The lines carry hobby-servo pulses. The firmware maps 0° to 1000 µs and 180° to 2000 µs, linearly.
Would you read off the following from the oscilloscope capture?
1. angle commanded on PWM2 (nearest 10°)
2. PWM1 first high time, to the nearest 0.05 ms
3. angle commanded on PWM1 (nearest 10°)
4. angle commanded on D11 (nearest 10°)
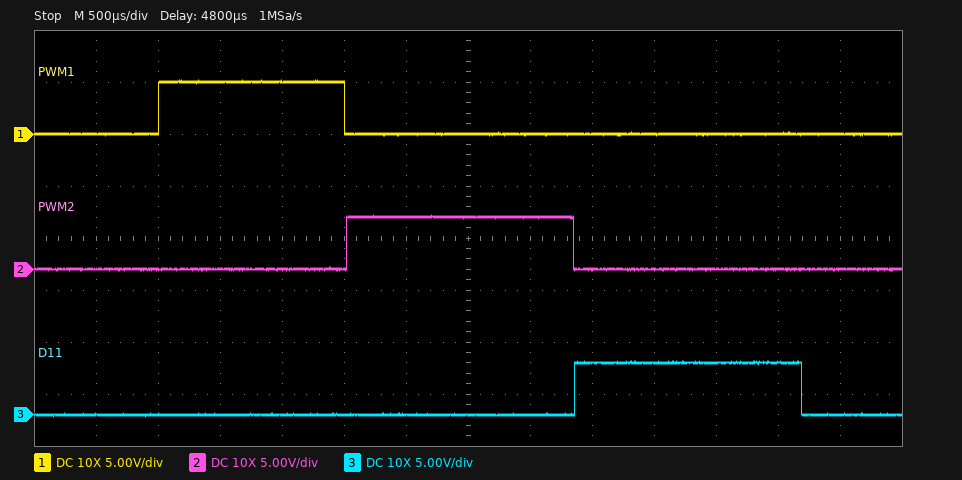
150°
1.50 ms
90°
150°
